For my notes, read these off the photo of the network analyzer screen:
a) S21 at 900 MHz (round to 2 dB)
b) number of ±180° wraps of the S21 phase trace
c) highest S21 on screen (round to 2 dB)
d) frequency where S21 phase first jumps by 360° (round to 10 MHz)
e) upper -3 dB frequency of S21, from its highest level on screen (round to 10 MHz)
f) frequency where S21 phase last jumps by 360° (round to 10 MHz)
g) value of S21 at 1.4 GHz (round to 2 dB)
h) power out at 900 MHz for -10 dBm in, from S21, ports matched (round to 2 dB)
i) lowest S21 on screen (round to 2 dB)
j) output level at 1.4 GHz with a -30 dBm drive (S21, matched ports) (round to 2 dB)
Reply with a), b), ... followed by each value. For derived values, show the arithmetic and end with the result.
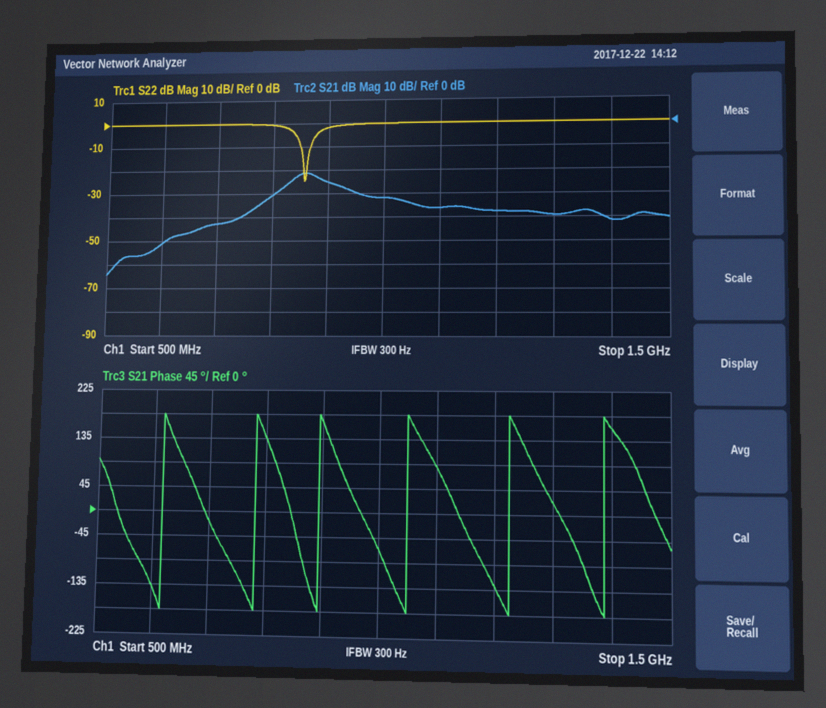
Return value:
a) -26 dB
b) 6
c) -22 dB
d) 620 MHz
e) 890 MHz
f) 1.39 GHz
g) -42 dB
h) -10 dBm + (-26 dB) = -36 dBm
i) -64 dB
j) -30 dBm + (-42 dB) = -72 dBm
